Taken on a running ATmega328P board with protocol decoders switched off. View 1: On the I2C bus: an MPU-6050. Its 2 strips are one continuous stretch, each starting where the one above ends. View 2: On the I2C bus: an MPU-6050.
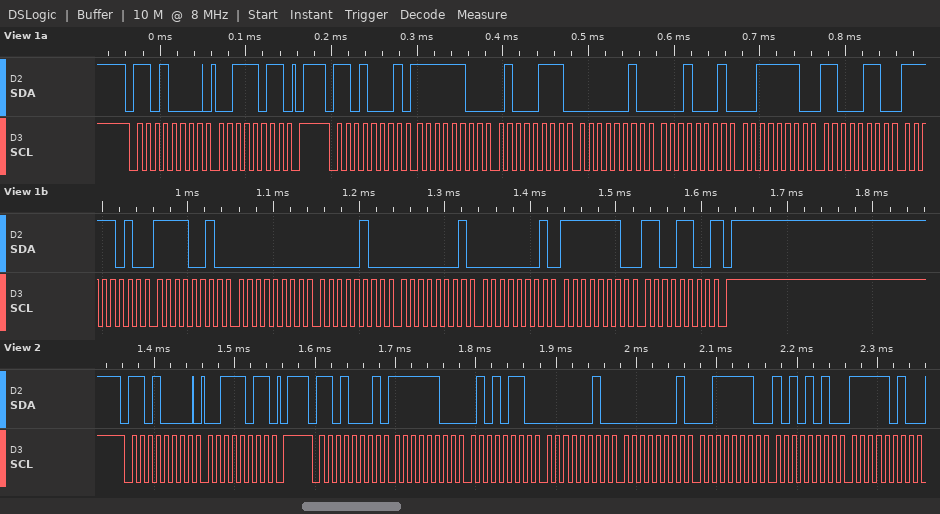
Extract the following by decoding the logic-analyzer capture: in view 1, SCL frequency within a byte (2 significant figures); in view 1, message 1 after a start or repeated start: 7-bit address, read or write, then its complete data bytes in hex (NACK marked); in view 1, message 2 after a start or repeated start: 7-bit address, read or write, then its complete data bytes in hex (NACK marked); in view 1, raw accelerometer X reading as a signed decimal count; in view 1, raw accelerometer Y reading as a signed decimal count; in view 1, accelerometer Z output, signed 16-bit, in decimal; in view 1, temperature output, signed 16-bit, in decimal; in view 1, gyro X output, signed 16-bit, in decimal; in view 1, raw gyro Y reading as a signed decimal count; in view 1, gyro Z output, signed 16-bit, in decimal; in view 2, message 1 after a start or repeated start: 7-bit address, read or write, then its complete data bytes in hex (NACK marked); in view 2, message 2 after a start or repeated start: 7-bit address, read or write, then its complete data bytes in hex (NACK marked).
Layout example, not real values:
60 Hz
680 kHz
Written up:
100 kHz
0x68 write: 3B
0x68 read: FC 47 02 11 3E C6 FA F2 00 04 01 01 FE CC NACK
-953
529
16070
-1294
4
257
-308
0x68 write: 3B
0x68 read: FC 56 02 01 3E AA FA
